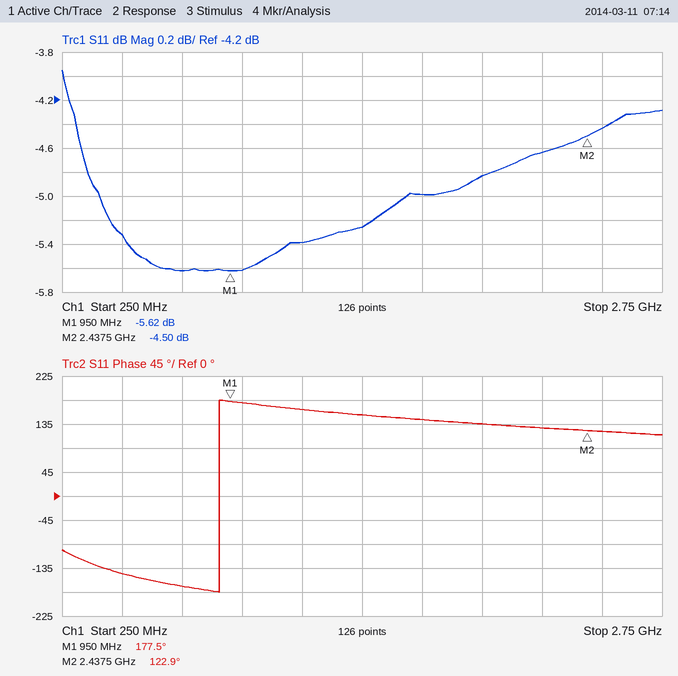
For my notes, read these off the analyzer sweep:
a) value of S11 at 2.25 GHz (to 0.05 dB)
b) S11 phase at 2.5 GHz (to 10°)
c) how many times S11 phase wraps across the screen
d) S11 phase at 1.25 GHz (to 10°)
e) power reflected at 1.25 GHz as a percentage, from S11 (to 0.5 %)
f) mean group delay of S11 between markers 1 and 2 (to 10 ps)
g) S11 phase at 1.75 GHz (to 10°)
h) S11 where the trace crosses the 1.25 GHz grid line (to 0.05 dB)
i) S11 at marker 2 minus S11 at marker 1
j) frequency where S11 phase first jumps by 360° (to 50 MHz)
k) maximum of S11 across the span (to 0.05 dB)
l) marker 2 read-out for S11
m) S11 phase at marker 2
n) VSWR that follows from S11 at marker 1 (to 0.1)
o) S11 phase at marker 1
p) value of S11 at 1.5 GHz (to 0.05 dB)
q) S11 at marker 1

-4.65 dB
120°
1
160°
29.0 %
100 ps
140°
-5.40 dB
1.12 dB
900 MHz
-3.95 dB
-4.50 dB
122.9°
3.2
177.5°
-5.25 dB
-5.62 dB
